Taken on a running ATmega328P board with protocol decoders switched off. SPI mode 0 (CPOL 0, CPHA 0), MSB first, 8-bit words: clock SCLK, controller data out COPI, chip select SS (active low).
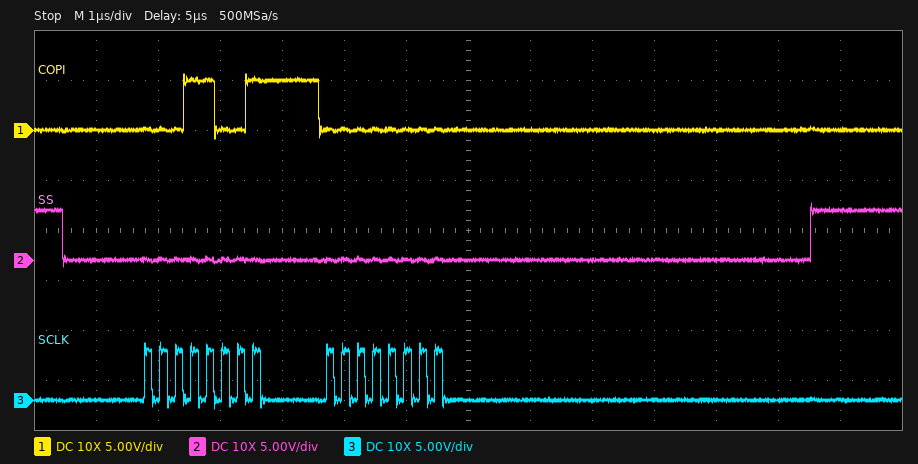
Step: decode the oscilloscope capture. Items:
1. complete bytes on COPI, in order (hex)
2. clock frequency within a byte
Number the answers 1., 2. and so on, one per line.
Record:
1. 19 00
2. 4 MHz
